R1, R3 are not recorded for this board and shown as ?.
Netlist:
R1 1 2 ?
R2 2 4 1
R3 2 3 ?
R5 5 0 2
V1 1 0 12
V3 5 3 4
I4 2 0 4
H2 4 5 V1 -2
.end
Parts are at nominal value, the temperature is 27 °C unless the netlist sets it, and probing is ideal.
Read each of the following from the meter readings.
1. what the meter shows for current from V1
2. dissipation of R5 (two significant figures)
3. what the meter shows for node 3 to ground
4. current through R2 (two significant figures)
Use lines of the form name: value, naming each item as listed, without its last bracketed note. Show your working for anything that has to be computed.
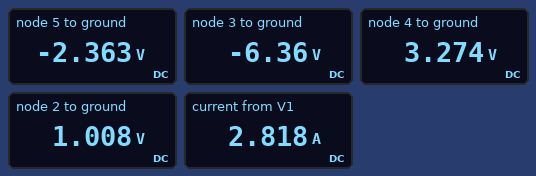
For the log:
what the meter shows for current from V1: 2.818 A
dissipation of R5: (0 V - (-2.363 V))^2 / 2 Ω = 2.8 W
what the meter shows for node 3 to ground: -6.36 V
current through R2: (3.274 V - 1.008 V) / 1 Ω = 2.3 A
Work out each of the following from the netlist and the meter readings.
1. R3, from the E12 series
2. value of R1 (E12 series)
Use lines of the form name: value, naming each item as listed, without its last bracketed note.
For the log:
R3, from the E12 series: 6.8 Ω
value of R1: 3.9 Ω
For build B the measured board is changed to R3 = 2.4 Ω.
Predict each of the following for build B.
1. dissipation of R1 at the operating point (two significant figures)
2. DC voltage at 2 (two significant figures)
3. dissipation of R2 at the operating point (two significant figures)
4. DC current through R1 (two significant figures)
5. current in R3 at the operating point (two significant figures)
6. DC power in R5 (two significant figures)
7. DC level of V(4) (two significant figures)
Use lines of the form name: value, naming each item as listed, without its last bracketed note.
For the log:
dissipation of R1 at the operating point: 35 W
DC voltage at 2: 330 mV
dissipation of R2 at the operating point: 13 W
DC current through R1: 3.0 A
current in R3 at the operating point: 2.6 A
DC power in R5: 2.0 W
DC level of V(4): 4.0 V
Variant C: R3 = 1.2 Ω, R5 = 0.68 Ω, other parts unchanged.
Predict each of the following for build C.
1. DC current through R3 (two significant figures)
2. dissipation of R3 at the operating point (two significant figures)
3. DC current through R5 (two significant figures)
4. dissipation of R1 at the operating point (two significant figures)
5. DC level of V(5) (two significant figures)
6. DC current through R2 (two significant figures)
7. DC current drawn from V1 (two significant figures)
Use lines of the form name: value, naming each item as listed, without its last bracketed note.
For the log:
DC current through R3: 4.1 A
dissipation of R3 at the operating point: 20 W
DC current through R5: 990 mA
dissipation of R1 at the operating point: 35 W
DC level of V(5): -670 mV
DC current through R2: 5.1 A
DC current drawn from V1: 3.0 A
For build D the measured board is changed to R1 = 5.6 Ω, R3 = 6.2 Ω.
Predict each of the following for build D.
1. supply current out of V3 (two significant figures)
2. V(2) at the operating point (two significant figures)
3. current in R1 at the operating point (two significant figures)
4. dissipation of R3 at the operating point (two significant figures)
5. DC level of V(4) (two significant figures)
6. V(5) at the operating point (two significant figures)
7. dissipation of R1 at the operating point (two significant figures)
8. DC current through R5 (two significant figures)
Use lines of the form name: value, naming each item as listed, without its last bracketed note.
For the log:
supply current out of V3: 980 mA
V(2) at the operating point: -1.2 V
current in R1 at the operating point: 2.4 A
dissipation of R3 at the operating point: 6.0 W
DC level of V(4): 1.4 V
V(5) at the operating point: -3.3 V
dissipation of R1 at the operating point: 31 W
DC current through R5: 1.6 A
